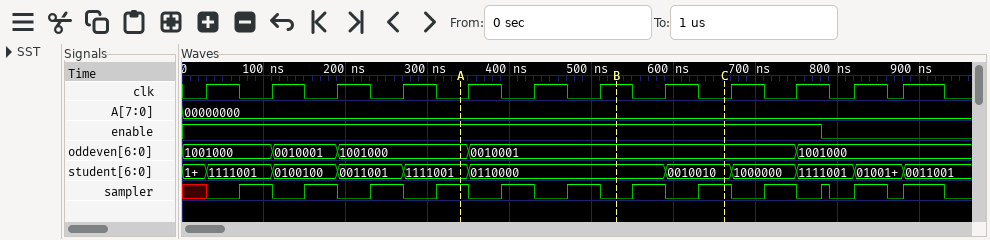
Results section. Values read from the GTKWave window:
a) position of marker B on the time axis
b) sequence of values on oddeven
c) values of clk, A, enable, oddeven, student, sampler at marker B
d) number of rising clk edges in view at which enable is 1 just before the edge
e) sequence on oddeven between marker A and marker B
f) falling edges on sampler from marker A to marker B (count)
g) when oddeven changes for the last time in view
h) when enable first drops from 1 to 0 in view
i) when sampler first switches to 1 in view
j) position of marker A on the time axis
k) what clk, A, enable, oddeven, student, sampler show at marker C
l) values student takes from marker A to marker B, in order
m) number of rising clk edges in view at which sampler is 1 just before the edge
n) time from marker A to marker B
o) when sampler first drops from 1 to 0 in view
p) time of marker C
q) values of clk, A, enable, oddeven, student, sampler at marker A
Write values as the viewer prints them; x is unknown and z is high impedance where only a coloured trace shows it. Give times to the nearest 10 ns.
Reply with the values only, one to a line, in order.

530 ns
1001000, 0010001, 1001000, 0010001, 1001000
clk=1, A=00000000, enable=1, oddeven=0010001, student=0110000, sampler=0
10
1001000, 0010001
3
750 ns
780 ns
70 ns
340 ns
clk=0, A=00000000, enable=1, oddeven=0010001, student=0010010, sampler=1
1111001, 0110000
9
190 ns
110 ns
660 ns
clk=0, A=00000000, enable=1, oddeven=1001000, student=1111001, sampler=1
